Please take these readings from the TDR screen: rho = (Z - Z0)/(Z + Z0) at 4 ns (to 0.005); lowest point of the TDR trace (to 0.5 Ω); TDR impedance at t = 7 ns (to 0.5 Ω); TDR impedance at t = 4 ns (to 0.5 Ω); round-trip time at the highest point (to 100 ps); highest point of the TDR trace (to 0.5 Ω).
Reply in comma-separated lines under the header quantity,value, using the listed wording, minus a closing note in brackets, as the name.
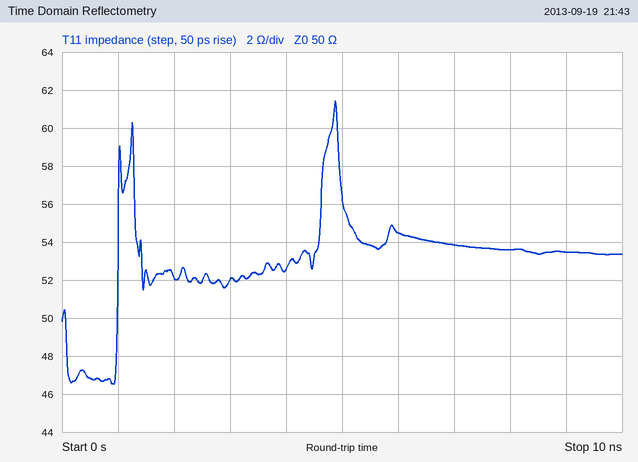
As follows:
quantity,value
rho = (Z - Z0)/(Z + Z0) at 4 ns,+0.025
lowest point of the TDR trace,46.5 Ω
TDR impedance at t = 7 ns,54.0 Ω
TDR impedance at t = 4 ns,52.5 Ω
round-trip time at the highest point,4.9 ns
highest point of the TDR trace,61.5 Ω
